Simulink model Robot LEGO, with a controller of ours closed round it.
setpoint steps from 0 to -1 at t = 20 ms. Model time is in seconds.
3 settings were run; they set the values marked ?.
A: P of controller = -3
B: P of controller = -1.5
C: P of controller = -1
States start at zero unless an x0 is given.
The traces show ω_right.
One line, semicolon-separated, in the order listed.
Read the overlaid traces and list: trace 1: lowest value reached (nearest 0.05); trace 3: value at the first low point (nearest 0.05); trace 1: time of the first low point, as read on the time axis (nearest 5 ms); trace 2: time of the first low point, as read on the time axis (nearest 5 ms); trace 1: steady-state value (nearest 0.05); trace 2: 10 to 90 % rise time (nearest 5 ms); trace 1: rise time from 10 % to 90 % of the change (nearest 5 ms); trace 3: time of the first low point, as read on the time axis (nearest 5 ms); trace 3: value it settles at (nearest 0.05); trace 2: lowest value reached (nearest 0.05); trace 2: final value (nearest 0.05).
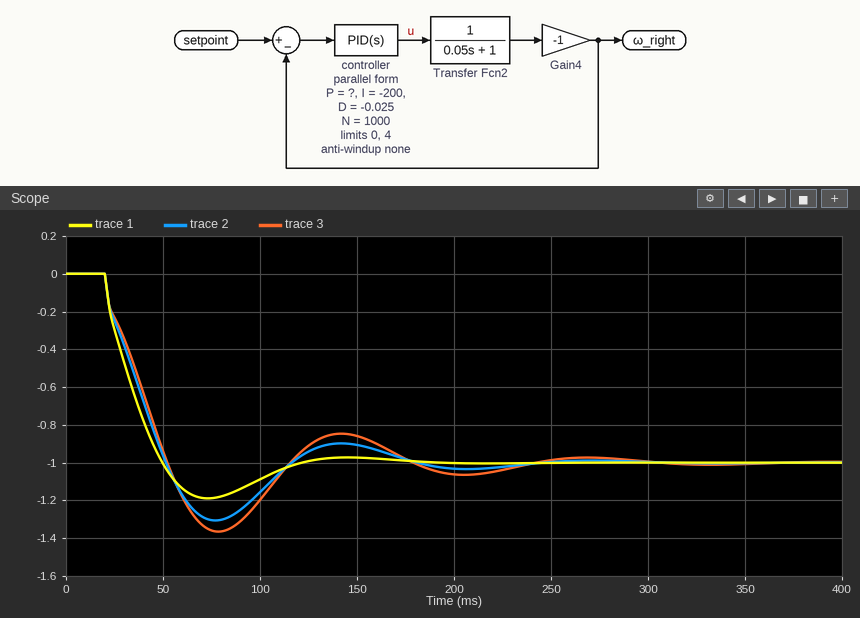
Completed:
-1.20; -1.35; 75 ms; 75 ms; -1.00; 25 ms; 25 ms; 80 ms; -1.00; -1.30; -1.00
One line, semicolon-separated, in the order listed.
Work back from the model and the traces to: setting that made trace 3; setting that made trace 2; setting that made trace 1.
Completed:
C; B; A
